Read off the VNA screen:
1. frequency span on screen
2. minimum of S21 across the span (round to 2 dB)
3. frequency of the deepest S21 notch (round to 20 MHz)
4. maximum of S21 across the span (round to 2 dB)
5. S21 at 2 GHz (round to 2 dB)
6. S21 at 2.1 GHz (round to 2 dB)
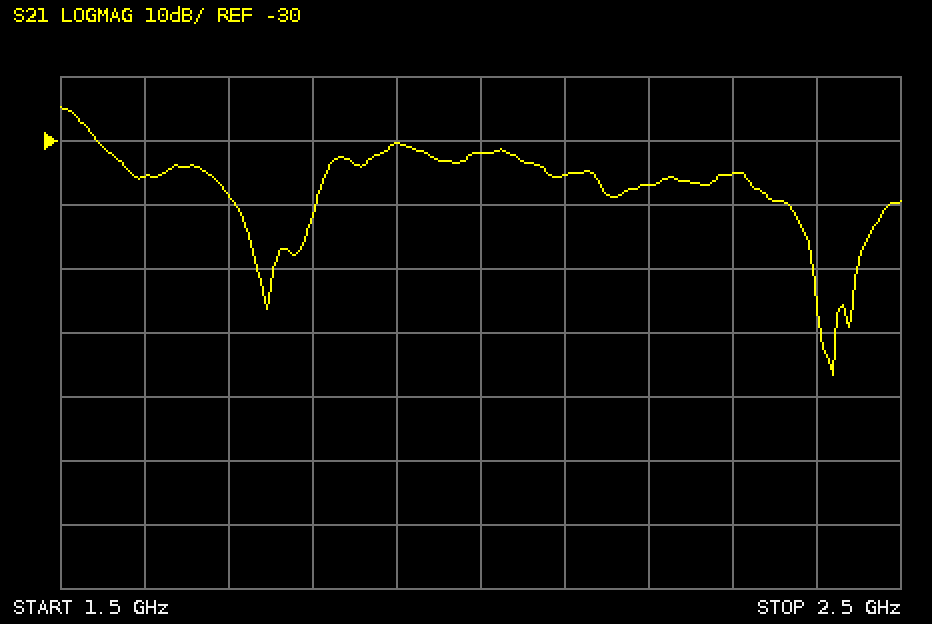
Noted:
1 GHz
-66 dB
2.42 GHz
-24 dB
-32 dB
-36 dB
